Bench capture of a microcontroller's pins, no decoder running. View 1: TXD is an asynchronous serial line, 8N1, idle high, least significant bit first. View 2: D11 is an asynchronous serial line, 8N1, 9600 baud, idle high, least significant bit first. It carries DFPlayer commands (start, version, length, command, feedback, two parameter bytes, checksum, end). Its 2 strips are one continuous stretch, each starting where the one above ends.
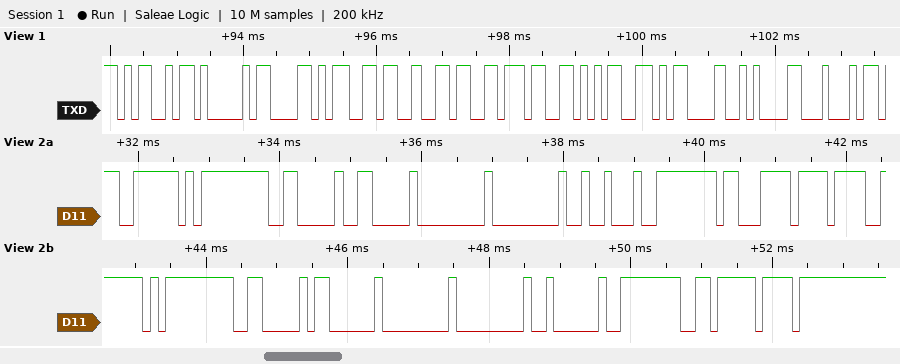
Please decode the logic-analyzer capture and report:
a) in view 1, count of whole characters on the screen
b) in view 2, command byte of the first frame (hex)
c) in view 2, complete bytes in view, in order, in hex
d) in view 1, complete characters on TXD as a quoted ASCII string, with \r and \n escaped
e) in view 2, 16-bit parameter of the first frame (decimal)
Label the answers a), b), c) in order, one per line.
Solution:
a) 10
b) 0x06
c) 0x7E 0xFF 0x06 0x06 0x00 0x00 0x12 0xFE 0xE3 0xEF 0x7E 0xFF 0x06 0x03 0x00 0x00 0x02 0xFE 0xF6 0xEF
d) "MAX6675\r\nD"
e) 18
